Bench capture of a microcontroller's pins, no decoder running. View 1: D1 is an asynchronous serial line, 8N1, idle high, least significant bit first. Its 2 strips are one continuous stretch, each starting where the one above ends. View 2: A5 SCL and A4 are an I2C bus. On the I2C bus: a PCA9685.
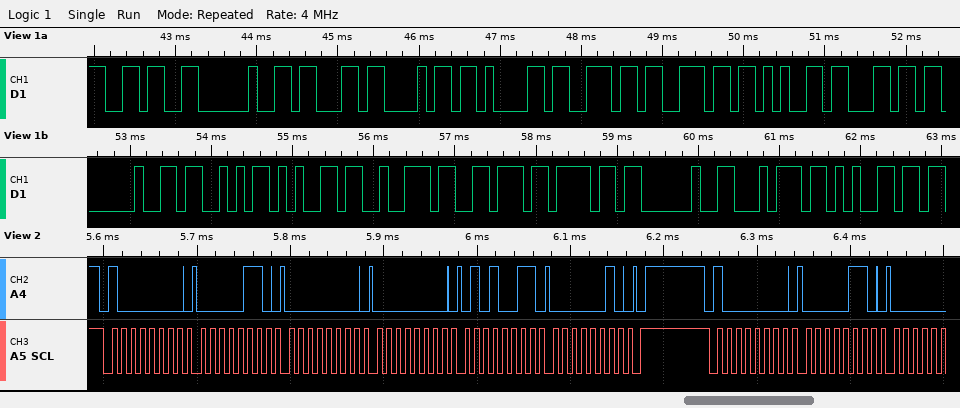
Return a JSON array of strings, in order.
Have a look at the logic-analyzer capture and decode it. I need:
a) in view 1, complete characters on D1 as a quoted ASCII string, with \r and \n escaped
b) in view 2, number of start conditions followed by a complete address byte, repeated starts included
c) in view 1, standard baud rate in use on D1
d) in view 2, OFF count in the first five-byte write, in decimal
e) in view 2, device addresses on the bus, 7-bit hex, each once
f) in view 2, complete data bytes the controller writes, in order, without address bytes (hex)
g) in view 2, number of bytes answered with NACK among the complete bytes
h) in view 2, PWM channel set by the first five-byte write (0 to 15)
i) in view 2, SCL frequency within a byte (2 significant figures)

["\"6 channel Servo te\"", "2", "9600 baud", "595", "0x40", "06 00 00 53 02 06", "0", "0", "100 kHz"]
